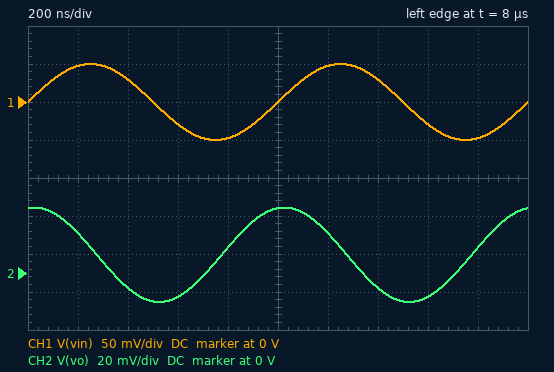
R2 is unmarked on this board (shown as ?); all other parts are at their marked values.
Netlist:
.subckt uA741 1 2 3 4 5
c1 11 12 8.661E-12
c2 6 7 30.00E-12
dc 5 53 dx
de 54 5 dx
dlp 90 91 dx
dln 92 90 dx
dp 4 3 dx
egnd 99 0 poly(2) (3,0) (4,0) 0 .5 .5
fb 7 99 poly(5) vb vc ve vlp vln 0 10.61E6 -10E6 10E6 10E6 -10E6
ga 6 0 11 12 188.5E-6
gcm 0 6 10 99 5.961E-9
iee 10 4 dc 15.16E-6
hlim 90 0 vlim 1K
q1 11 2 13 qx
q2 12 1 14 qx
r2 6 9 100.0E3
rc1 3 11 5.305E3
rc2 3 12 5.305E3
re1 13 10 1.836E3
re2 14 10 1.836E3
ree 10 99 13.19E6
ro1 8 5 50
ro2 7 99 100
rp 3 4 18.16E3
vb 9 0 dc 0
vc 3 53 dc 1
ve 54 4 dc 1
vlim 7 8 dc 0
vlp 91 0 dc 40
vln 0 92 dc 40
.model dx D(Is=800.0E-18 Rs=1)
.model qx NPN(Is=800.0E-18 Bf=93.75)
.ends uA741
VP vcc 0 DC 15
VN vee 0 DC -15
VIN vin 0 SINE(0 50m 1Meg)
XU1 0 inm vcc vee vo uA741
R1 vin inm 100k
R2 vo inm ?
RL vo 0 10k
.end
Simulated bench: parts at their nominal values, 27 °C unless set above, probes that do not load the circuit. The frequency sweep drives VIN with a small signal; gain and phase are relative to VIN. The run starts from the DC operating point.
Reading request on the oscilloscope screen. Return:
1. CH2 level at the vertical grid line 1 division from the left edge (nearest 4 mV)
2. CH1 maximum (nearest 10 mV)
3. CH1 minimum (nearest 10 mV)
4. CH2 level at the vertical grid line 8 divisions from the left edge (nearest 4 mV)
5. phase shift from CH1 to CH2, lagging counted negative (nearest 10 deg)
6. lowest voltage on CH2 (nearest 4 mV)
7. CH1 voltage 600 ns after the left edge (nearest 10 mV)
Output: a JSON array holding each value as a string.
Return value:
["20 mV", "50 mV", "-50 mV", "-12 mV", "80 deg", "-16 mV", "-30 mV"]
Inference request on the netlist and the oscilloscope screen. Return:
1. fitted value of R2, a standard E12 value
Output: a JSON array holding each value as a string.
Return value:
["120 kΩ"]
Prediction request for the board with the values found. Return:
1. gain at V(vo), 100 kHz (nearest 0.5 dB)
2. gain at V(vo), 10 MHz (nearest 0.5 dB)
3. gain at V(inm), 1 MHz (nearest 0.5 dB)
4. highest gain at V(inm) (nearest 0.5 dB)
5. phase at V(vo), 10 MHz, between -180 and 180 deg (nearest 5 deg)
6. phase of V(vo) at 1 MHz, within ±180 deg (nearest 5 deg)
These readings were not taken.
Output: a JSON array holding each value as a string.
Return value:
["1.5 dB", "-41.0 dB", "-4.5 dB", "-4.5 dB", "10 deg", "80 deg"]
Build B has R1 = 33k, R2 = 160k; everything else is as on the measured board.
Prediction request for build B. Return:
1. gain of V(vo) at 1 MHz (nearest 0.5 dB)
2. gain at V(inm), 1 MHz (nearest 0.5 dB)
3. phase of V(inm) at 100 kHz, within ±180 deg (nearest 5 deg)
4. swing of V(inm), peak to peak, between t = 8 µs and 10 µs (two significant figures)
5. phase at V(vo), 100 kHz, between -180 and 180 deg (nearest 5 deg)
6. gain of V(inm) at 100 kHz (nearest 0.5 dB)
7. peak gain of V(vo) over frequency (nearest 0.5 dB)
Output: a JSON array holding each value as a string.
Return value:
["-2.5 dB", "-1.5 dB", "60 deg", "86 mV", "150 deg", "-7.5 dB", "13.5 dB"]
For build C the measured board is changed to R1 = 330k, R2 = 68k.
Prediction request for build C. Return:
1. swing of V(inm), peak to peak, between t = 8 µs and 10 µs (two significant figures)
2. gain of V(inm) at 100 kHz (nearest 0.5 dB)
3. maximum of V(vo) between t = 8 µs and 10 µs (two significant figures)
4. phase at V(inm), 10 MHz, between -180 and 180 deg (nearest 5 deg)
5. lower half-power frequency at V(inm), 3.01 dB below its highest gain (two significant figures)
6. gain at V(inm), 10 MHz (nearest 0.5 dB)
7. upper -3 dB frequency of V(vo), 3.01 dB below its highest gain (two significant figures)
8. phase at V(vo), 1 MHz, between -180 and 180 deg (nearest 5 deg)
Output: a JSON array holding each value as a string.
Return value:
["18 mV", "-33.5 dB", "13 mV", "0 deg", "700 kHz", "-15.5 dB", "1.1 MHz", "100 deg"]
